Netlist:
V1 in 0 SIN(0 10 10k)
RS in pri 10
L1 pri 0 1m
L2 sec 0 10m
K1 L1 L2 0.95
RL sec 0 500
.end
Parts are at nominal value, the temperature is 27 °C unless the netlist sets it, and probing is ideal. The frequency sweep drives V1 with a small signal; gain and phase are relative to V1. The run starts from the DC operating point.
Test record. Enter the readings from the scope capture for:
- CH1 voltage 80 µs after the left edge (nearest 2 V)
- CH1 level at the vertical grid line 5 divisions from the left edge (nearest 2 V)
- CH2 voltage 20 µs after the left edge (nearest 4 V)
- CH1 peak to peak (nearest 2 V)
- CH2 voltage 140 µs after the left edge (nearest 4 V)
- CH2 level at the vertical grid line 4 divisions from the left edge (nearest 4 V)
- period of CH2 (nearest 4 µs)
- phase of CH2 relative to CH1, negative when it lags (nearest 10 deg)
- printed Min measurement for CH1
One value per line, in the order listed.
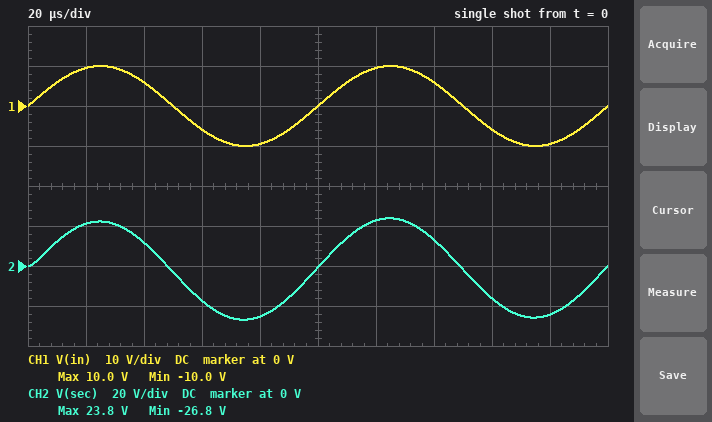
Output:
-10 V
0 V
20 V
20 V
12 V
-24 V
100 µs
0 deg
-10.0 V
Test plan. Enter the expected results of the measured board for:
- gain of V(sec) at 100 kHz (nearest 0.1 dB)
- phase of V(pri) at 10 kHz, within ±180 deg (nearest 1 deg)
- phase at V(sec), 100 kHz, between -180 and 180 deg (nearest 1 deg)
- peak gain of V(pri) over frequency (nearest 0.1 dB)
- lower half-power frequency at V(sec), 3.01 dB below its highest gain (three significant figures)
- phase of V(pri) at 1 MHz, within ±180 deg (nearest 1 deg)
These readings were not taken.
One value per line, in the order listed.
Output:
4.9 dB
9 deg
-45 deg
0 dB
1.31 kHz
1 deg
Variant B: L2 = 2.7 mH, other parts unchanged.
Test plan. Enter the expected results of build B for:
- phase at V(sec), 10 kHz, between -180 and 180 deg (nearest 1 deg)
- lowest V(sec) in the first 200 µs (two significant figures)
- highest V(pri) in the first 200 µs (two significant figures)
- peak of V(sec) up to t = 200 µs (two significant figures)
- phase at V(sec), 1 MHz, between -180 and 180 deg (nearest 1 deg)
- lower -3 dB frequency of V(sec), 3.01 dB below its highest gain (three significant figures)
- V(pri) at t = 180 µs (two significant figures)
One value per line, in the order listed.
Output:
7 deg
-16 V
9.0 V
14 V
-72 deg
1.50 kHz
-8.7 V
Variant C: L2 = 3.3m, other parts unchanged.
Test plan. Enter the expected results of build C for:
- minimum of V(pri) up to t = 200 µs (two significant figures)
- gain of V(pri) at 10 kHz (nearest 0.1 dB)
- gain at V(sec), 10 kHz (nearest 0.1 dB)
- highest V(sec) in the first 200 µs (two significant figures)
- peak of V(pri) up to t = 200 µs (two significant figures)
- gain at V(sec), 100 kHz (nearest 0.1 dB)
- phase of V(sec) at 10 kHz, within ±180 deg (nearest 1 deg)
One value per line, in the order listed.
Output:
-10 V
-0.6 dB
4.1 dB
15 V
8.9 V
3.6 dB
6 deg
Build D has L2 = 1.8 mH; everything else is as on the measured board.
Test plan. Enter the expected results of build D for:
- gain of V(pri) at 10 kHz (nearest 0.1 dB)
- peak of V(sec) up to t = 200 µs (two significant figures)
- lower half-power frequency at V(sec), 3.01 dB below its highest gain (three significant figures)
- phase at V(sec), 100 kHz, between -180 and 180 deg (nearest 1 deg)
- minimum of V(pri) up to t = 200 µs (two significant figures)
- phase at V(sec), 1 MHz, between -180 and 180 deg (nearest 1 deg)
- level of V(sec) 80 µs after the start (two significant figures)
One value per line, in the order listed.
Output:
-0.4 dB
12 V
1.53 kHz
-11 deg
-10 V
-65 deg
-12 V
